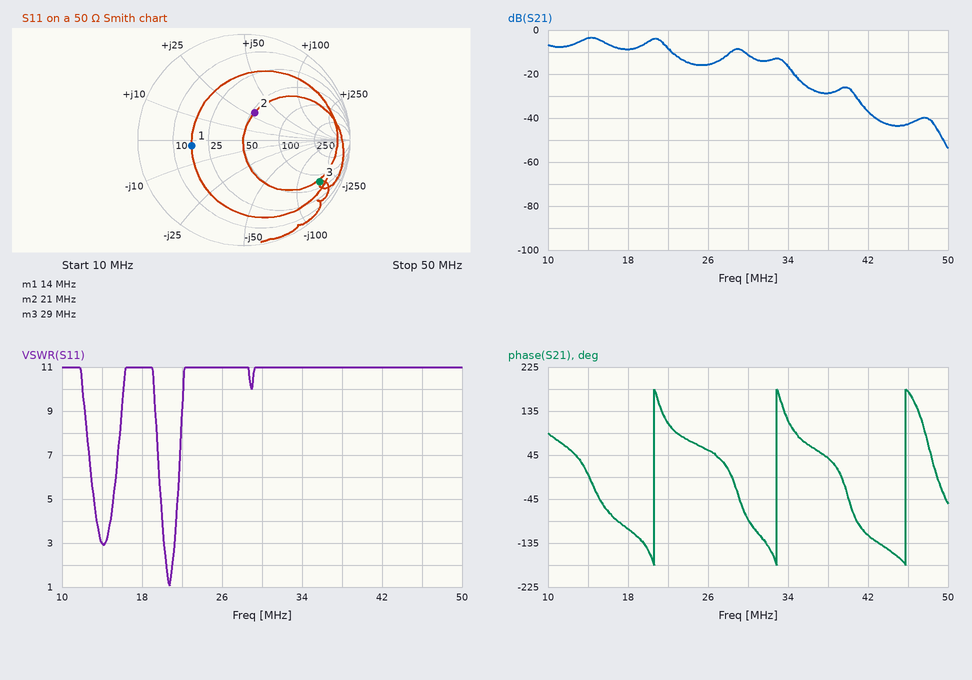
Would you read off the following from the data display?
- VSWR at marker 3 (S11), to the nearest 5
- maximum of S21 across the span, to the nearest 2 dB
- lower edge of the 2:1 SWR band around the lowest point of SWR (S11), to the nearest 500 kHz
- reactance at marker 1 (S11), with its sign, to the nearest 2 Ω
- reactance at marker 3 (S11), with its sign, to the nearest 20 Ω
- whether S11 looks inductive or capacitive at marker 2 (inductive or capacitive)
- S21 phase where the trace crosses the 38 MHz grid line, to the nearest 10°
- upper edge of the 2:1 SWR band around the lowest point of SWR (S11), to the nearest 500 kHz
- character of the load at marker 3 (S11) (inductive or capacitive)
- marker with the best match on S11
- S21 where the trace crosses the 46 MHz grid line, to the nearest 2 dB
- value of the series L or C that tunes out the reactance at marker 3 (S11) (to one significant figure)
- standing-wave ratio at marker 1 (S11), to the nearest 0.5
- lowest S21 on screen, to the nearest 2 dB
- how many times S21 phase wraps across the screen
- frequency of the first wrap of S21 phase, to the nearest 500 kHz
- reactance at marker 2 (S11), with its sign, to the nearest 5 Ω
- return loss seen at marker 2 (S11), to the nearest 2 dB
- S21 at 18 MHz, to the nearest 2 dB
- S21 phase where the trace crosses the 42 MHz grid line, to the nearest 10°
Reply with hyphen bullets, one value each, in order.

- 10
- -4 dB
- 20.5 MHz
- -2 Ω
- -160 Ω
- inductive
- 40°
- 21.0 MHz
- capacitive
- marker 2
- -42 dB
- 900 nH
- 3.0
- -54 dB
- 3
- 20.5 MHz
- +30 Ω
- 12 dB
- -8 dB
- -120°
